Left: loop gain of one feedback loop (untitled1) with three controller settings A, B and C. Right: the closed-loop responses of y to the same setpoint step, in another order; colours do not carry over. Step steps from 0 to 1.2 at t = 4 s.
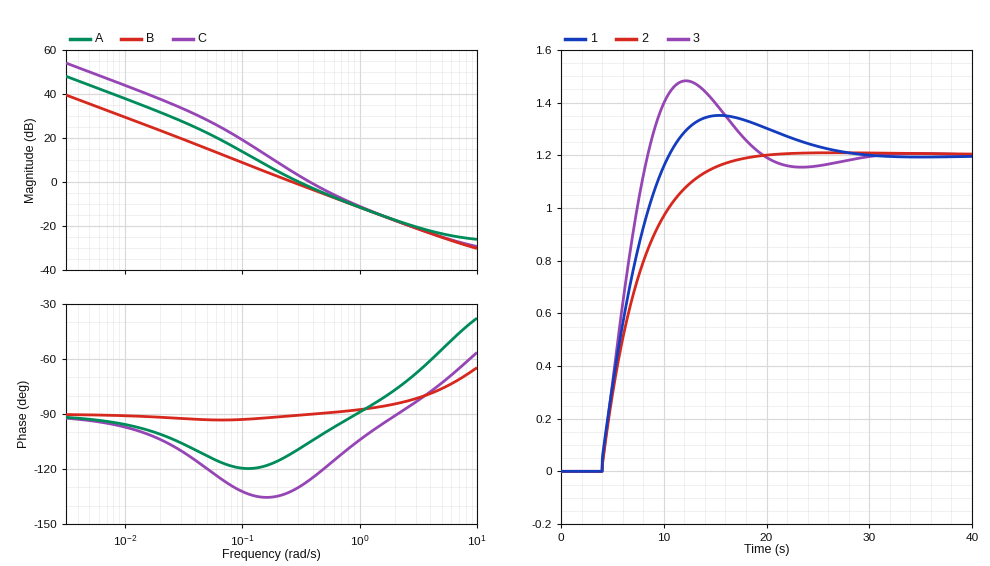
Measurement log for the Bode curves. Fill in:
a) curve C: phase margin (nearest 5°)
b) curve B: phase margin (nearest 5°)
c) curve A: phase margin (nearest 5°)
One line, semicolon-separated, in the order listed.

55°; 90°; 70°
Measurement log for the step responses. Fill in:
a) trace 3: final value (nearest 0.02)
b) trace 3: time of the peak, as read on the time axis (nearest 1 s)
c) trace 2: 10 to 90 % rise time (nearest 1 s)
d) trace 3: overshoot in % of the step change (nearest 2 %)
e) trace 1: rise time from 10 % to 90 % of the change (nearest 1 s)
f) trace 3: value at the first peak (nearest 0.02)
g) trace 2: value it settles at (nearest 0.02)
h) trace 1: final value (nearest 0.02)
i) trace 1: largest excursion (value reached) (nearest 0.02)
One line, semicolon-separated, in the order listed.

1.20; 12 s; 8 s; 24 %; 5 s; 1.48; 1.20; 1.20; 1.36
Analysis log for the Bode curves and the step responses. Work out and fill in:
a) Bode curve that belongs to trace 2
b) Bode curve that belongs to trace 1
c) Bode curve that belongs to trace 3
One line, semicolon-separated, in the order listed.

B; A; C
